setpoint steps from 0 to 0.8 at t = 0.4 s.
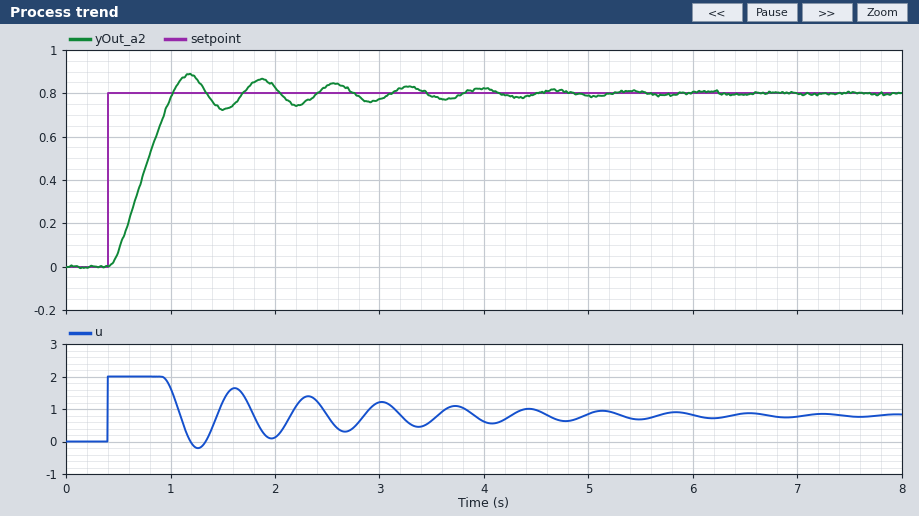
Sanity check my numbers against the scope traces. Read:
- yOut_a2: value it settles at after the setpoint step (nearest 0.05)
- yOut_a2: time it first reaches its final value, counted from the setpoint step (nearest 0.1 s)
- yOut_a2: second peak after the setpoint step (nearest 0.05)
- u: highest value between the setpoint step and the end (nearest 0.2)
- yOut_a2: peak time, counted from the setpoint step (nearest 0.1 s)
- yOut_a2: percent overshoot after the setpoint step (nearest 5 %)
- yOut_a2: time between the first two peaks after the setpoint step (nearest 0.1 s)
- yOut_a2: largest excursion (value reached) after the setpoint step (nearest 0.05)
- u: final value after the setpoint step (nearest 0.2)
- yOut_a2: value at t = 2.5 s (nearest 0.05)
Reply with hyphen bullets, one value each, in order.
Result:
- 0.80
- 0.6 s
- 0.85
- 2.0
- 0.8 s
- 10 %
- 0.7 s
- 0.90
- 0.8
- 0.85
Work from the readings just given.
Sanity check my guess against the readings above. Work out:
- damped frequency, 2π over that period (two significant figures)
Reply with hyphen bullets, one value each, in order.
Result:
- 9.0 rad/s
